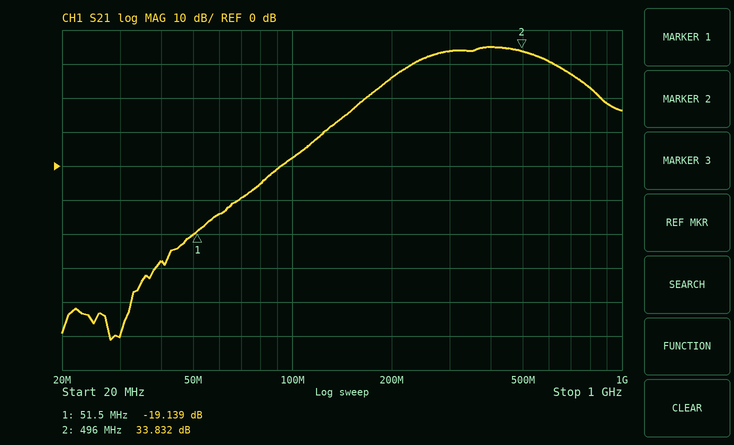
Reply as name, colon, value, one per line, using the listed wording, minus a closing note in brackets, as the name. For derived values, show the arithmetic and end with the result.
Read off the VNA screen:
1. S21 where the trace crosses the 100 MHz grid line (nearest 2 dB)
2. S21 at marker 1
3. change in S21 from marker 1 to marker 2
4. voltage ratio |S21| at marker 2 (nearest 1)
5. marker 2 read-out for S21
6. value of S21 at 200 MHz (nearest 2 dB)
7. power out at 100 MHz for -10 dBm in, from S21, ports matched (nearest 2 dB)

S21 where the trace crosses the 100 MHz grid line: 2 dB
S21 at marker 1: -19.139 dB
change in S21 from marker 1 to marker 2: 33.832 − (-19.139) = 52.971 dB
voltage ratio |S21| at marker 2: 10^(33.832/20) ≈ 49
marker 2 read-out for S21: 33.832 dB
value of S21 at 200 MHz: 26 dB
power out at 100 MHz for -10 dBm in, from S21, ports matched: -10 dBm + (2 dB) = -8 dBm
